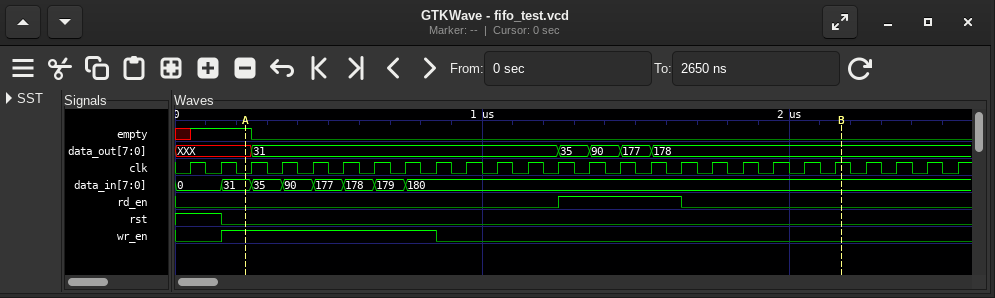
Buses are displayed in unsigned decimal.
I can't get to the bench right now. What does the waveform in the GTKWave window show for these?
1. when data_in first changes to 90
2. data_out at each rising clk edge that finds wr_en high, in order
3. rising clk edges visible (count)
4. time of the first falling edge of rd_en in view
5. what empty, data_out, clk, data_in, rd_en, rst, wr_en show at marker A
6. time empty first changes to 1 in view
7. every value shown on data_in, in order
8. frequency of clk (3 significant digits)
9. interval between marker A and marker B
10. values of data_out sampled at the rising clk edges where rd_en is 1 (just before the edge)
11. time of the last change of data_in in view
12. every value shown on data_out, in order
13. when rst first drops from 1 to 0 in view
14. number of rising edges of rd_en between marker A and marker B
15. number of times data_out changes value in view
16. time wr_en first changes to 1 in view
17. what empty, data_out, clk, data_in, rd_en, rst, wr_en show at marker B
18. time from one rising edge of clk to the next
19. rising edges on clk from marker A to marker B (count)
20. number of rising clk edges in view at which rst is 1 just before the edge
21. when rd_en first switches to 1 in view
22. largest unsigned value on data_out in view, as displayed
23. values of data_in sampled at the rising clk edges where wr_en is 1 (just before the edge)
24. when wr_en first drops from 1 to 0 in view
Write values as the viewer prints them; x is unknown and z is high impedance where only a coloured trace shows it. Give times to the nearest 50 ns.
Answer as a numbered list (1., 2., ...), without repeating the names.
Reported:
1. 350 ns
2. XXX, 31, 31, 31, 31, 31, 31
3. 26
4. 1650 ns
5. empty=1, data_out=XXX, clk=0, data_in=31, rd_en=0, rst=0, wr_en=1
6. 50 ns
7. 0, 31, 35, 90, 177, 178, 179, 180
8. 10.0 MHz
9. 1950 ns
10. 35, 90, 177, 178
11. 750 ns
12. XXX, 31, 35, 90, 177, 178
13. 150 ns
14. 1
15. 5
16. 150 ns
17. empty=0, data_out=178, clk=1, data_in=180, rd_en=0, rst=0, wr_en=0
18. 100 ns
19. 20
20. 2
21. 1250 ns
22. 178
23. 31, 35, 90, 177, 178, 179, 180
24. 850 ns
